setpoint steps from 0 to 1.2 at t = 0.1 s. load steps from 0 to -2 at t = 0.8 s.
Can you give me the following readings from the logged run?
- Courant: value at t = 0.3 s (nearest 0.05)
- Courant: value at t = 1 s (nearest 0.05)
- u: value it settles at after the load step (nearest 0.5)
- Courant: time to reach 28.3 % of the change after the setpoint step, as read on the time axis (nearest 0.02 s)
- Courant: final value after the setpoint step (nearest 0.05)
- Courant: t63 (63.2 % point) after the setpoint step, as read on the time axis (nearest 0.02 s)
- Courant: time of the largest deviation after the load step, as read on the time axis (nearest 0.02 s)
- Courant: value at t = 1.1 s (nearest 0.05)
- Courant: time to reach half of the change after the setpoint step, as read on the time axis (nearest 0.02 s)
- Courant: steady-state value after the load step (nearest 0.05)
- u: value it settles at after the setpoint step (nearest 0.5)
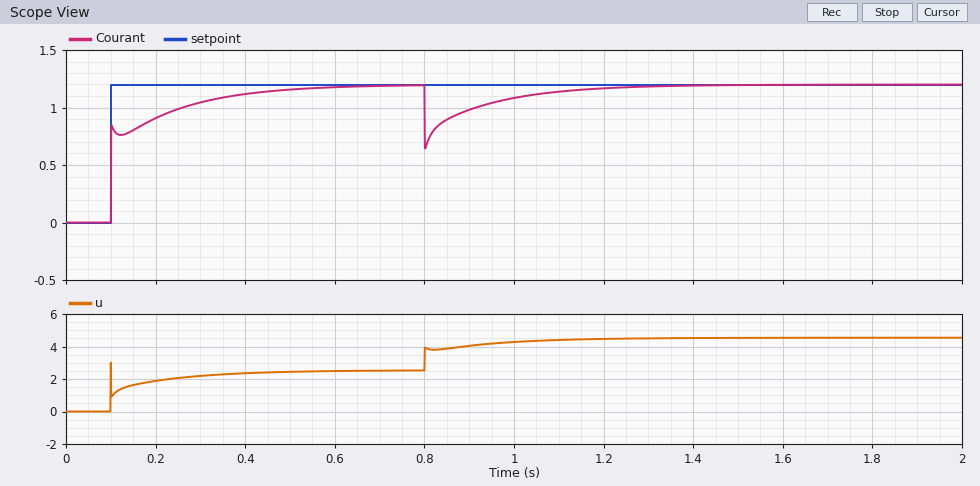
1.05
1.10
4.5
0.10 s
1.20
0.10 s
0.80 s
1.15
0.10 s
1.20
2.5
